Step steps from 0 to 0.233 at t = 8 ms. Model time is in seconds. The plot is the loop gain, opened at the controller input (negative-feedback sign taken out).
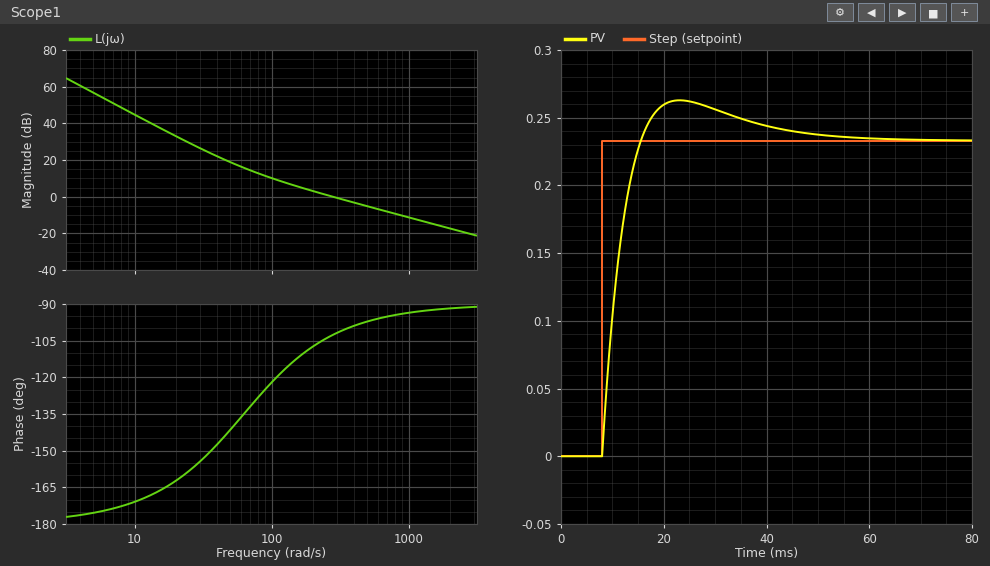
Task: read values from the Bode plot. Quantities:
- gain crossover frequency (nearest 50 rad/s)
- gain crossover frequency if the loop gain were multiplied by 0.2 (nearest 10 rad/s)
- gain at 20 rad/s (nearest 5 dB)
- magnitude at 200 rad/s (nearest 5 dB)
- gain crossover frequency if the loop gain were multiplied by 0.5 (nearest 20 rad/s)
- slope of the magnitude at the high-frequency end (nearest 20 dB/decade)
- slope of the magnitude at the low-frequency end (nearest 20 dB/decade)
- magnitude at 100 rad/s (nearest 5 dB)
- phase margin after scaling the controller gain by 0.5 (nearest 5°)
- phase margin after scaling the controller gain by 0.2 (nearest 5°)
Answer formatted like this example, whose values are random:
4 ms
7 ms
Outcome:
300 rad/s
70 rad/s
35 dB
5 dB
140 rad/s
-20 dB/decade
-40 dB/decade
10 dB
65°
50°
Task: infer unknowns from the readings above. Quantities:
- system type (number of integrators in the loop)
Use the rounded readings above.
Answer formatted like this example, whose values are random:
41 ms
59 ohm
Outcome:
2
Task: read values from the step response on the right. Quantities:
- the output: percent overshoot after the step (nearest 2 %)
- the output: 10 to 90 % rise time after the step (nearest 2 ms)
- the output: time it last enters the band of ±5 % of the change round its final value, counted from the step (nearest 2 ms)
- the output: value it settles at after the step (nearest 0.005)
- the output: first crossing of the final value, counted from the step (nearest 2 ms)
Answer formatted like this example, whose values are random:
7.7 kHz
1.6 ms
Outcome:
12 %
6 ms
32 ms
0.235
8 ms
